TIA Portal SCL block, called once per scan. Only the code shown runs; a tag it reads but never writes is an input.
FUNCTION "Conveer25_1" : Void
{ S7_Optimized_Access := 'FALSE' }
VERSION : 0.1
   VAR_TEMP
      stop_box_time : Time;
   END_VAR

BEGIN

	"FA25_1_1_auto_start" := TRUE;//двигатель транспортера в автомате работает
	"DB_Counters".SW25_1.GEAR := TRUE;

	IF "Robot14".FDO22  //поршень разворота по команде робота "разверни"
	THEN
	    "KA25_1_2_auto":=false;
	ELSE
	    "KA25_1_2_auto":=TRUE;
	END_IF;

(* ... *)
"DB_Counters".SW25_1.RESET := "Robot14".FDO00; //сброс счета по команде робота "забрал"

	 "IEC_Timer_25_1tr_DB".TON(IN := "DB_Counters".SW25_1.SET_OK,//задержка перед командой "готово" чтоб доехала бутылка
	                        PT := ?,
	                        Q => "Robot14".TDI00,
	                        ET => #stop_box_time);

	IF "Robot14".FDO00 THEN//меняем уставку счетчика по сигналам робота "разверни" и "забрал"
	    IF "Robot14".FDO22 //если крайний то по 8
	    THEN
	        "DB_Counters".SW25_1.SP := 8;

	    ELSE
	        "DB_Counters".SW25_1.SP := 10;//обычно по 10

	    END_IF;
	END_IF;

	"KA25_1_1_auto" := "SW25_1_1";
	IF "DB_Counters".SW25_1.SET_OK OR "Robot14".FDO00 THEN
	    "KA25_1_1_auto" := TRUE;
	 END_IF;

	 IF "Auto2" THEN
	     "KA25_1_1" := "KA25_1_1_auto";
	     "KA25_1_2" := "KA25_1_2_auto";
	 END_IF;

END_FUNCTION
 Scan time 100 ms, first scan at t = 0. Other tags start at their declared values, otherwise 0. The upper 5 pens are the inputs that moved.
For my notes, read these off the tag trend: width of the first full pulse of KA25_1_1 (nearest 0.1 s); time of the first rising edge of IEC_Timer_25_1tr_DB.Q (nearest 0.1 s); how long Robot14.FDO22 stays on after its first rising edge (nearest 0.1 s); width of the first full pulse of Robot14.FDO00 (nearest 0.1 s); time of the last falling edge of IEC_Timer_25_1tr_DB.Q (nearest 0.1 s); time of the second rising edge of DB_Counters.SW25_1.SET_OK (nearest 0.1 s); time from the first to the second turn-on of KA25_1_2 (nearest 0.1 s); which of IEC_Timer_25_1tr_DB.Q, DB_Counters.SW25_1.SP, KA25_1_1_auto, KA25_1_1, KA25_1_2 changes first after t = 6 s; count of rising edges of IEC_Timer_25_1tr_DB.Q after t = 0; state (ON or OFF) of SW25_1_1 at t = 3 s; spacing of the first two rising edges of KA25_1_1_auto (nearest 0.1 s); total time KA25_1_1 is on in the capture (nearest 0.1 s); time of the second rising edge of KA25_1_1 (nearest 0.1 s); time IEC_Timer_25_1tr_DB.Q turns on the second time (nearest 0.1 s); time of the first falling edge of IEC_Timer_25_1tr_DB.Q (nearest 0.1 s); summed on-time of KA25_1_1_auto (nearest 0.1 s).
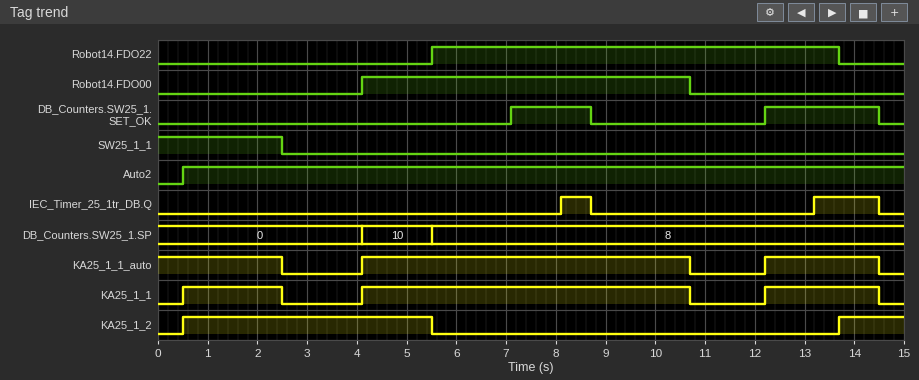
2.0 s
8.1 s
8.2 s
6.6 s
14.5 s
12.2 s
13.2 s
IEC_Timer_25_1tr_DB.Q
2
OFF
8.1 s
10.9 s
4.1 s
13.2 s
8.7 s
11.4 s
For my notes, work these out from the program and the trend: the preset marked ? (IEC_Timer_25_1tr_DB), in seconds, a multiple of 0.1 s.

1.0 s
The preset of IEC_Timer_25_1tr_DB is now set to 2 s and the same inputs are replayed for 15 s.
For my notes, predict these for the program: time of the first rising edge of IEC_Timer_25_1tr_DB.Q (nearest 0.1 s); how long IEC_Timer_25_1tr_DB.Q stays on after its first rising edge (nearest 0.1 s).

14.2 s
0.3 s
